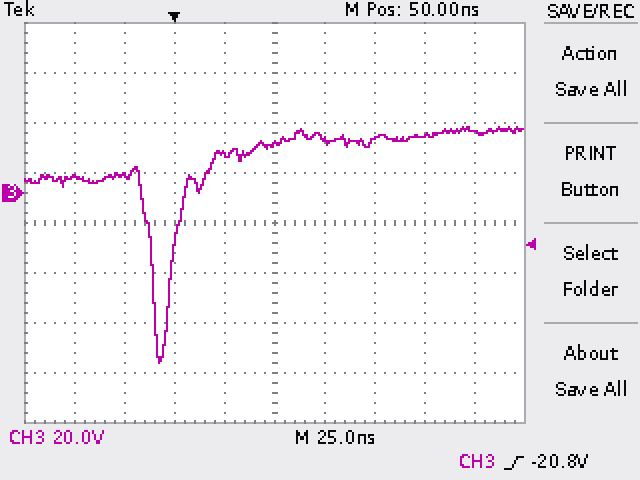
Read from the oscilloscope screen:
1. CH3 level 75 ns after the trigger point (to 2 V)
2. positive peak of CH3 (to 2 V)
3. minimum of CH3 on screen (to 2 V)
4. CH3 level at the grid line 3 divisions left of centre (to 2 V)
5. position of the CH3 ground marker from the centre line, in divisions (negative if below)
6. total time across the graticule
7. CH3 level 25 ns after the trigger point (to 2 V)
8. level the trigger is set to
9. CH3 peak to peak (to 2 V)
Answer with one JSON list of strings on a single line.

["22 V", "26 V", "-68 V", "6 V", "+0.6 div", "250 ns", "16 V", "-20.8 V", "94 V"]
